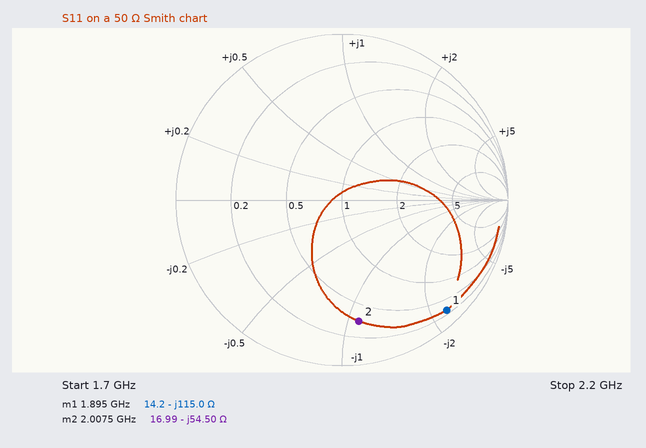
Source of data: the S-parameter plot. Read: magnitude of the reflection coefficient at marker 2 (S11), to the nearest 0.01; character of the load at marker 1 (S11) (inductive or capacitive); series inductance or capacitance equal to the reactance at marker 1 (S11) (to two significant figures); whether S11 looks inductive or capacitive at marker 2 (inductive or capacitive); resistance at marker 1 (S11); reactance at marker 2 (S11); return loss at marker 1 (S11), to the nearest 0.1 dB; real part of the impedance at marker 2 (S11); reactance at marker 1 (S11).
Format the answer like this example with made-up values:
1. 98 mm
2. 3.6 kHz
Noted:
1. 0.74
2. capacitive
3. 730 fF
4. capacitive
5. 14.2 Ω
6. -54.50 Ω
7. 0.8 dB
8. 16.99 Ω
9. -115.0 Ω
